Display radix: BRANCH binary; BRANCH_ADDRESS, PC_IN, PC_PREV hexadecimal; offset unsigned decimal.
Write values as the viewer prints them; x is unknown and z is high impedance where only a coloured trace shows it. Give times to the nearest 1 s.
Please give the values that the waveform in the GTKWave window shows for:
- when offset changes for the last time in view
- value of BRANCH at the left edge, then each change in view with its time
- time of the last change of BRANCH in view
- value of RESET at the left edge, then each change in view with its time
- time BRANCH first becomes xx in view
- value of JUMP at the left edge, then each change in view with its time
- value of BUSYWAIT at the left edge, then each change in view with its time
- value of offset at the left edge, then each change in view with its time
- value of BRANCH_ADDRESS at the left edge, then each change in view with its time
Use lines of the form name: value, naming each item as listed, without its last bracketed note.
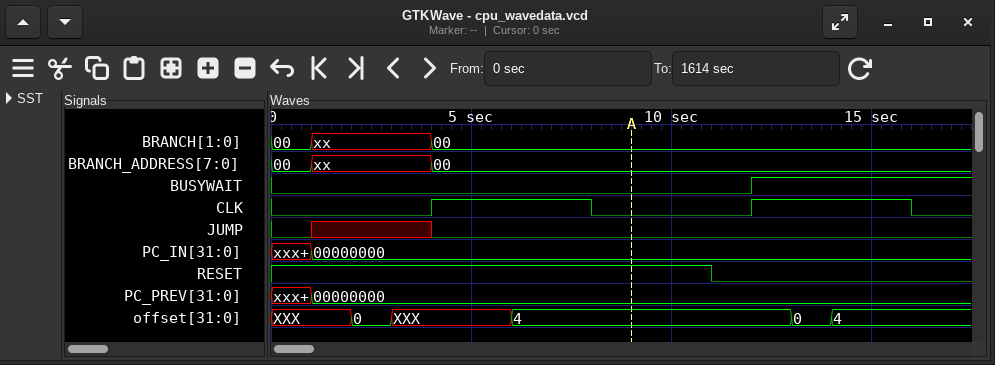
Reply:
when offset changes for the last time in view: 14 s
value of BRANCH at the left edge, then each change in view with its time: 00, xx at 1 s, 00 at 4 s
time of the last change of BRANCH in view: 4 s
value of RESET at the left edge, then each change in view with its time: 1, 0 at 11 s
time BRANCH first becomes xx in view: 1 s
value of JUMP at the left edge, then each change in view with its time: 0, x at 1 s, 0 at 4 s
value of BUSYWAIT at the left edge, then each change in view with its time: 0, 1 at 12 s
value of offset at the left edge, then each change in view with its time: XXX, 0 at 2 s, XXX at 3 s, 4 at 6 s, 0 at 13 s, 4 at 14 s
value of BRANCH_ADDRESS at the left edge, then each change in view with its time: 00, xx at 1 s, 00 at 4 s
